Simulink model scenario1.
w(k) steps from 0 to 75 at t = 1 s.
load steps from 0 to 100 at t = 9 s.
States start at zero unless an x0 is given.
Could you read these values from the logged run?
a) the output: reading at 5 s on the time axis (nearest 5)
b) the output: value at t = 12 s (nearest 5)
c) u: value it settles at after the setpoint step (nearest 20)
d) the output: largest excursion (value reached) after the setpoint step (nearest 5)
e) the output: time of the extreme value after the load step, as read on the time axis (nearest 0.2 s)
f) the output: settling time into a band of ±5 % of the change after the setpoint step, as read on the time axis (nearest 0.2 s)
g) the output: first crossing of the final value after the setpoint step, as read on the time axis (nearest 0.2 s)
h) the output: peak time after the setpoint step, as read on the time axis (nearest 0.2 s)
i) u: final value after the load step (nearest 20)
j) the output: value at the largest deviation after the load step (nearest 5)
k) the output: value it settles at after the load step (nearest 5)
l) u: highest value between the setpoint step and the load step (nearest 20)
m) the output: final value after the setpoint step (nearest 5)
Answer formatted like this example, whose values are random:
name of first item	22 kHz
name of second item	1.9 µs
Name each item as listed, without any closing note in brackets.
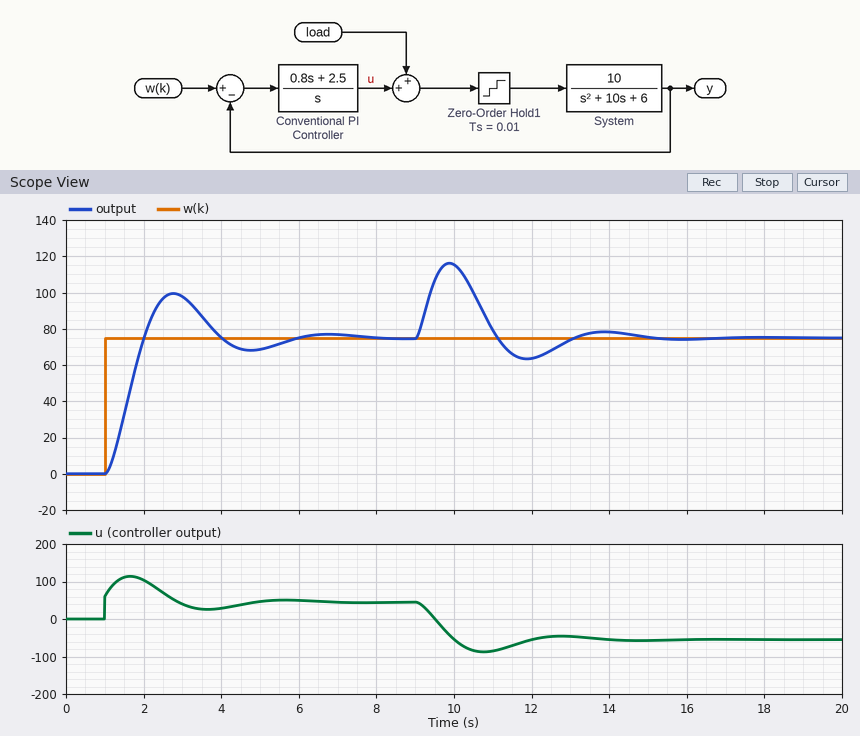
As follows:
the output: reading at 5 s on the time axis	70
the output: value at t = 12 s	65
u: value it settles at after the setpoint step	40
the output: largest excursion (value reached) after the setpoint step	100
the output: time of the extreme value after the load step, as read on the time axis	9.8 s
the output: settling time into a band of ±5 % of the change after the setpoint step, as read on the time axis	5.4 s
the output: first crossing of the final value after the setpoint step, as read on the time axis	2.0 s
the output: peak time after the setpoint step, as read on the time axis	2.8 s
u: final value after the load step	-60
the output: value at the largest deviation after the load step	115
the output: value it settles at after the load step	75
u: highest value between the setpoint step and the load step	120
the output: final value after the setpoint step	75
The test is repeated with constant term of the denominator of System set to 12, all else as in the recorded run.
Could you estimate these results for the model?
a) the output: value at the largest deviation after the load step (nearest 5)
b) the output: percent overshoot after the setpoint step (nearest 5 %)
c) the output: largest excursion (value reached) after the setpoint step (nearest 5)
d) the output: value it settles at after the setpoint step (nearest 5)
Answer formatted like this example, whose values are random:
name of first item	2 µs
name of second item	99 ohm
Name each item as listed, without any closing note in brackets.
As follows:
the output: value at the largest deviation after the load step	110
the output: percent overshoot after the setpoint step	10 %
the output: largest excursion (value reached) after the setpoint step	85
the output: value it settles at after the setpoint step	75
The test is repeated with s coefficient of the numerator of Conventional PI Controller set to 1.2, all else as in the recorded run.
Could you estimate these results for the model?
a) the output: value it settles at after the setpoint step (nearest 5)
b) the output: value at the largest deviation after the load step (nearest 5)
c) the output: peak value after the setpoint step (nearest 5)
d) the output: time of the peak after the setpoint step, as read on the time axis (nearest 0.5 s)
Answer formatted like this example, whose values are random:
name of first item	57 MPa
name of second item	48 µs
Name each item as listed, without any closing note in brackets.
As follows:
the output: value it settles at after the setpoint step	75
the output: value at the largest deviation after the load step	110
the output: peak value after the setpoint step	90
the output: time of the peak after the setpoint step, as read on the time axis	2.5 s
